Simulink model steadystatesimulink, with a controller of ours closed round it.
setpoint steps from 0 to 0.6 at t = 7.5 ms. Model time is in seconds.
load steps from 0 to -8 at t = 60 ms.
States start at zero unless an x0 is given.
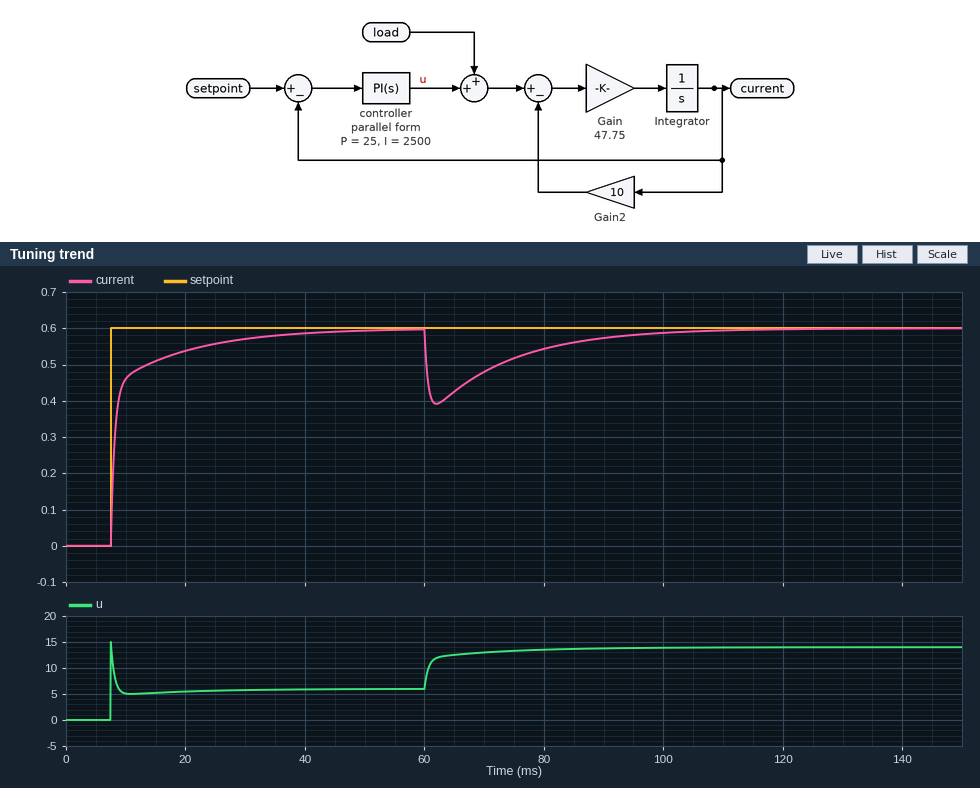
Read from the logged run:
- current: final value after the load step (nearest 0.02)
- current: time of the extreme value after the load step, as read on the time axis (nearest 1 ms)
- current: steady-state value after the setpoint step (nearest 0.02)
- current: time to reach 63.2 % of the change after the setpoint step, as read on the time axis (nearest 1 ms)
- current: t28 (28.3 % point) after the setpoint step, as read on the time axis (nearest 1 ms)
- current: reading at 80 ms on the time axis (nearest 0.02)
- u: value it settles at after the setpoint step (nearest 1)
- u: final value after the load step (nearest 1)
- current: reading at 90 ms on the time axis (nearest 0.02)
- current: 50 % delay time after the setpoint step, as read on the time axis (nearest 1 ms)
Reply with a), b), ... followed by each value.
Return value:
a) 0.60
b) 62 ms
c) 0.60
d) 9 ms
e) 8 ms
f) 0.54
g) 6
h) 14
i) 0.58
j) 8 ms
